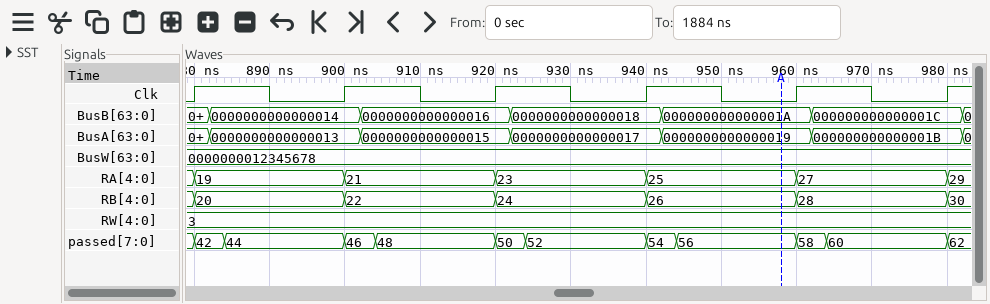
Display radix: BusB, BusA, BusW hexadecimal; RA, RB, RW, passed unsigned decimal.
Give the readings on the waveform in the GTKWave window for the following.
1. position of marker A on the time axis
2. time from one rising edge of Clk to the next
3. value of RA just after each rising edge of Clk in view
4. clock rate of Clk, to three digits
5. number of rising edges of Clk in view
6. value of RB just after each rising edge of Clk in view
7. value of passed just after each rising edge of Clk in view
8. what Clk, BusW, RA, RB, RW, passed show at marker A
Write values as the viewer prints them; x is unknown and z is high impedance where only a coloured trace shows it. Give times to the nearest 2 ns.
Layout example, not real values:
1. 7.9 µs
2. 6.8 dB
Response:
1. 958 ns
2. 20 ns
3. 19, 21, 23, 25, 27, 29
4. 50.0 MHz
5. 6
6. 20, 22, 24, 26, 28, 30
7. 42, 46, 50, 54, 58, 62
8. Clk=0, BusW=0000000012345678, RA=25, RB=26, RW=3, passed=56
